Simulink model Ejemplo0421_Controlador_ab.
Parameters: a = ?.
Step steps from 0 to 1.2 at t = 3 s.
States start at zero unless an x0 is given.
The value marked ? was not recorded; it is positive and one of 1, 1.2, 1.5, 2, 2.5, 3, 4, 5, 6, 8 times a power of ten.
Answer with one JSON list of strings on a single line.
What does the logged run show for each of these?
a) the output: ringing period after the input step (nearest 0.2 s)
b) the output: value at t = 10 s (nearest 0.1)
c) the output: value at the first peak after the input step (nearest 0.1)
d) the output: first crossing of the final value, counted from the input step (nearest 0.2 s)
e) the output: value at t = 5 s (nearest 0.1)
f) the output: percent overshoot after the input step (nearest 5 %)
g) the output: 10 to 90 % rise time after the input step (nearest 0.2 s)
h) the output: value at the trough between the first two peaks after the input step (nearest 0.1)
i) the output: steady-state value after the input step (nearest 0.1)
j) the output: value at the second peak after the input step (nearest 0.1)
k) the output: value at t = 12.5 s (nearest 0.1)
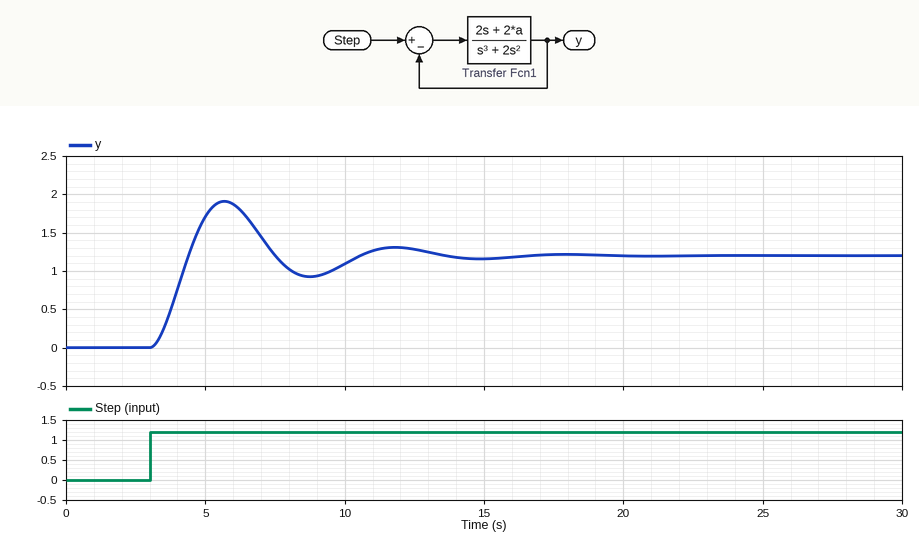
["6.2 s", "1.1", "1.9", "1.4 s", "1.7", "60 %", "1.0 s", "0.9", "1.2", "1.3", "1.3"]
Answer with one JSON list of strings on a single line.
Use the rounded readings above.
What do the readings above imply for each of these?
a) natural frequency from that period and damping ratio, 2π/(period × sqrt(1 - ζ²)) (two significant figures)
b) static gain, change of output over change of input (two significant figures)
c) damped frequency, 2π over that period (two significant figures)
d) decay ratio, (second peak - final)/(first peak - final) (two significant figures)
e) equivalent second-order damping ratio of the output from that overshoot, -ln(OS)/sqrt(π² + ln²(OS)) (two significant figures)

["1.0 rad/s", "1.0", "1.0 rad/s", "0.14", "0.16"]
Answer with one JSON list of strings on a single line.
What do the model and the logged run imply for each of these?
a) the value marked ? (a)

["0.8"]
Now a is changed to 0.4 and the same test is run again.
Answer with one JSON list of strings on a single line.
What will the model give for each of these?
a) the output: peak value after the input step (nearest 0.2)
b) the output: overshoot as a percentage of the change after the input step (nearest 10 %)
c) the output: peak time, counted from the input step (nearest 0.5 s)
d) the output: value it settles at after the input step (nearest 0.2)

["1.6", "40 %", "3.0 s", "1.2"]
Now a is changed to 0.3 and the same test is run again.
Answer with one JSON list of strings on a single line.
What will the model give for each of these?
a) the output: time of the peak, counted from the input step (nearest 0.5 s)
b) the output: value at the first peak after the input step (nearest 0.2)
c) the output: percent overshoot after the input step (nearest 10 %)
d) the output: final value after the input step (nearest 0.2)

["3.0 s", "1.6", "30 %", "1.2"]
